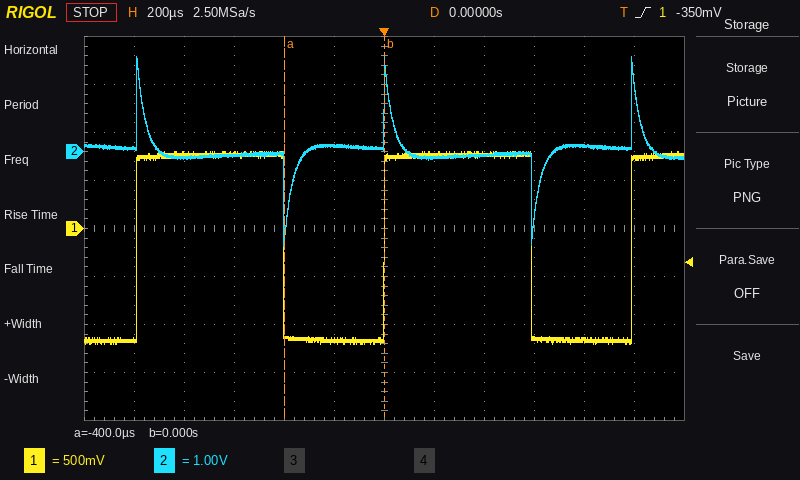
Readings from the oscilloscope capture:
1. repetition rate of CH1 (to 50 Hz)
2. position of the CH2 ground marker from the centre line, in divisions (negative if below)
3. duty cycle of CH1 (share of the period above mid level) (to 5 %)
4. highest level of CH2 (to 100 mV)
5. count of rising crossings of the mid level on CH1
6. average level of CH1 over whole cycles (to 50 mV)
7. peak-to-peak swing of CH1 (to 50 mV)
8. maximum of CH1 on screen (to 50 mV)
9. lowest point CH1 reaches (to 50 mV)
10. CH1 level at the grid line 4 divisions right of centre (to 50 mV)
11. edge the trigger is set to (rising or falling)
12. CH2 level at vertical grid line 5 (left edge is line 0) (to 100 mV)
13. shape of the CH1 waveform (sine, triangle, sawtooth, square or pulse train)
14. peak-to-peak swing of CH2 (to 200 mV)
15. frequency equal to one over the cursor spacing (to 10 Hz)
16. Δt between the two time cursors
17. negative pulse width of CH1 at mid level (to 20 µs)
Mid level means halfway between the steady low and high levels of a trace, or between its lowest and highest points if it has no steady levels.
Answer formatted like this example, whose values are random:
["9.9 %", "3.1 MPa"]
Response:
["1.00 kHz", "+1.6 div", "60 %", "2.0 V", "3", "0 mV", "2.00 V", "800 mV", "-1.20 V", "-1.15 V", "rising", "100 mV", "pulse train", "4.0 V", "2.50 kHz", "400 µs", "400 µs"]
